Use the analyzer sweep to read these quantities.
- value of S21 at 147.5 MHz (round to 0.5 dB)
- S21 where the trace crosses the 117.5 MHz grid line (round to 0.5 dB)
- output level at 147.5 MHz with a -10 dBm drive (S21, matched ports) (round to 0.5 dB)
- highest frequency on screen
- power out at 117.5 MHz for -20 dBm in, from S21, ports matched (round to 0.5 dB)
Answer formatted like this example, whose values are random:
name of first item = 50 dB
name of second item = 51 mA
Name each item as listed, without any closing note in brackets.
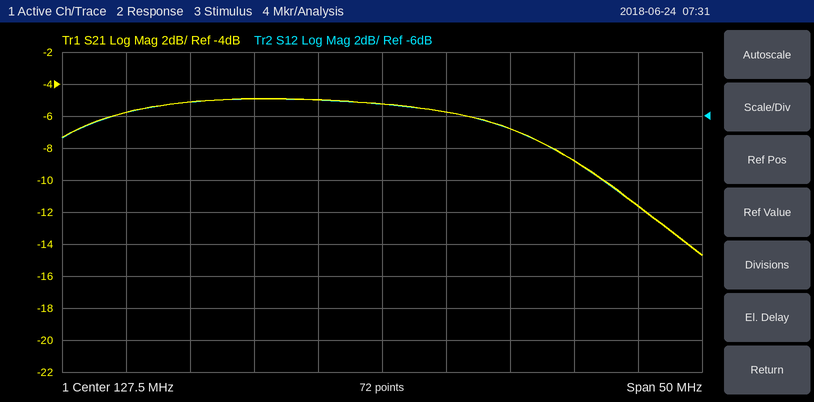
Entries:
value of S21 at 147.5 MHz = -11.5 dB
S21 where the trace crosses the 117.5 MHz grid line = -5.0 dB
output level at 147.5 MHz with a -10 dBm drive (S21, matched ports) = -21.5 dBm
highest frequency on screen = 152.5 MHz
power out at 117.5 MHz for -20 dBm in, from S21, ports matched = -25.0 dBm
